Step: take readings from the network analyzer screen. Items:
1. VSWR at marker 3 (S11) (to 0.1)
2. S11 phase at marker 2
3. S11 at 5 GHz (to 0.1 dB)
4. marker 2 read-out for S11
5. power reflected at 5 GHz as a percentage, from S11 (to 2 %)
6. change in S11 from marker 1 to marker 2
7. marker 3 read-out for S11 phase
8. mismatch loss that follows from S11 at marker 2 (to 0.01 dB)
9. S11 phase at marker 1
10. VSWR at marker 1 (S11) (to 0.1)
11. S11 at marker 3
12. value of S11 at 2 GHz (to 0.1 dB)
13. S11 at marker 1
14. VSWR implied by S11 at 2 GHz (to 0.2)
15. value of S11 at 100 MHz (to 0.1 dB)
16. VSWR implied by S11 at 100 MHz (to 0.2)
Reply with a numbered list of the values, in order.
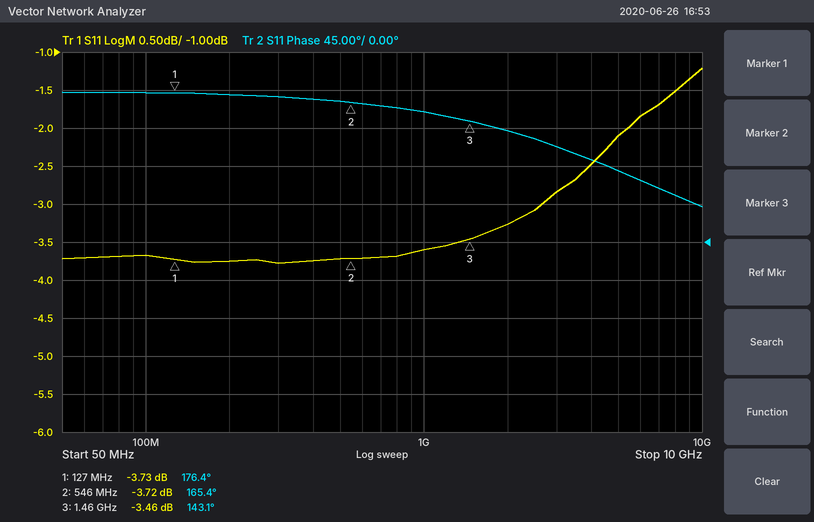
1. 5.1
2. 165.4°
3. -2.1 dB
4. -3.72 dB
5. 62 %
6. 0.01 dB
7. 143.1°
8. 2.40 dB
9. 176.4°
10. 4.7
11. -3.46 dB
12. -3.3 dB
13. -3.73 dB
14. 5.4
15. -3.7 dB
16. 4.8
